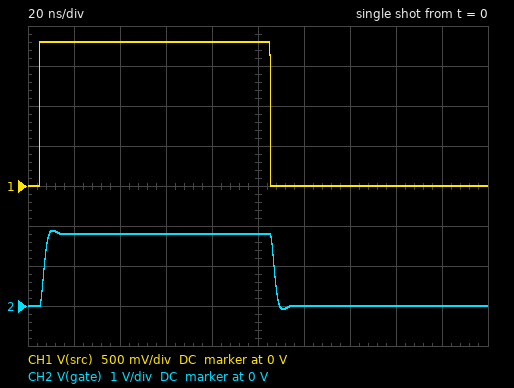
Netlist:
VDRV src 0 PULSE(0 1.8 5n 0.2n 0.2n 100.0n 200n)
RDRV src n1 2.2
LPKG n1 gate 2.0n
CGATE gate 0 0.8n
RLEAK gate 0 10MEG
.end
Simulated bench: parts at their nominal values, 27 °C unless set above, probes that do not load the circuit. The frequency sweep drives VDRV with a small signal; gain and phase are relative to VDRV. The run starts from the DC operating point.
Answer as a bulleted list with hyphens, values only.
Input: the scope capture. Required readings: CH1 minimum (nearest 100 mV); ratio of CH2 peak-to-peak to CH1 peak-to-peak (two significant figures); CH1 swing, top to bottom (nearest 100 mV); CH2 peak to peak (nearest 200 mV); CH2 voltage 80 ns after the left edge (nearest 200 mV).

- 0 V
- 1.1
- 1.8 V
- 2.0 V
- 1.8 V
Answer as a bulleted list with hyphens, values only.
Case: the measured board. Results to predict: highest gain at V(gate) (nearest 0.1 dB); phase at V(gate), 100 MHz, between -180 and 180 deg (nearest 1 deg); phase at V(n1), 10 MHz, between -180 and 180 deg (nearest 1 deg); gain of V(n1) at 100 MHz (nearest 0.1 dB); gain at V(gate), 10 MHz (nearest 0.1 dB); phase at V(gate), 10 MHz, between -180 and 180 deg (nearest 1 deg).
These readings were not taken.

- 0 dB
- -72 deg
- -6 deg
- -10.0 dB
- 0 dB
- -6 deg
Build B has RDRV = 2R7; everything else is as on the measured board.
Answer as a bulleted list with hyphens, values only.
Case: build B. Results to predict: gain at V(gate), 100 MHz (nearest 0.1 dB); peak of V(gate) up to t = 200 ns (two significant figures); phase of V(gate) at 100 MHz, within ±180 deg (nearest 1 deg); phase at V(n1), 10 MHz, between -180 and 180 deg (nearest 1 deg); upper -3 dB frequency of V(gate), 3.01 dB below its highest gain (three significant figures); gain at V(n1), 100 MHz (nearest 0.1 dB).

- -3.0 dB
- 1.8 V
- -75 deg
- -8 deg
- 101 MHz
- -11.6 dB
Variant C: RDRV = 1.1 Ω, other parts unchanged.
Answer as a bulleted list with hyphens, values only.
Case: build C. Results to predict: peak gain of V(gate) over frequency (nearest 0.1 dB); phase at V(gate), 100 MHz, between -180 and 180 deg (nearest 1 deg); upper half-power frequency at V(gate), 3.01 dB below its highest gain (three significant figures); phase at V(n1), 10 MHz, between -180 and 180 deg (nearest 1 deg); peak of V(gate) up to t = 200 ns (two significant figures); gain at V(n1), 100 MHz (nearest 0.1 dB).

- 3.7 dB
- -56 deg
- 149 MHz
- -3 deg
- 2.4 V
- -5.1 dB
